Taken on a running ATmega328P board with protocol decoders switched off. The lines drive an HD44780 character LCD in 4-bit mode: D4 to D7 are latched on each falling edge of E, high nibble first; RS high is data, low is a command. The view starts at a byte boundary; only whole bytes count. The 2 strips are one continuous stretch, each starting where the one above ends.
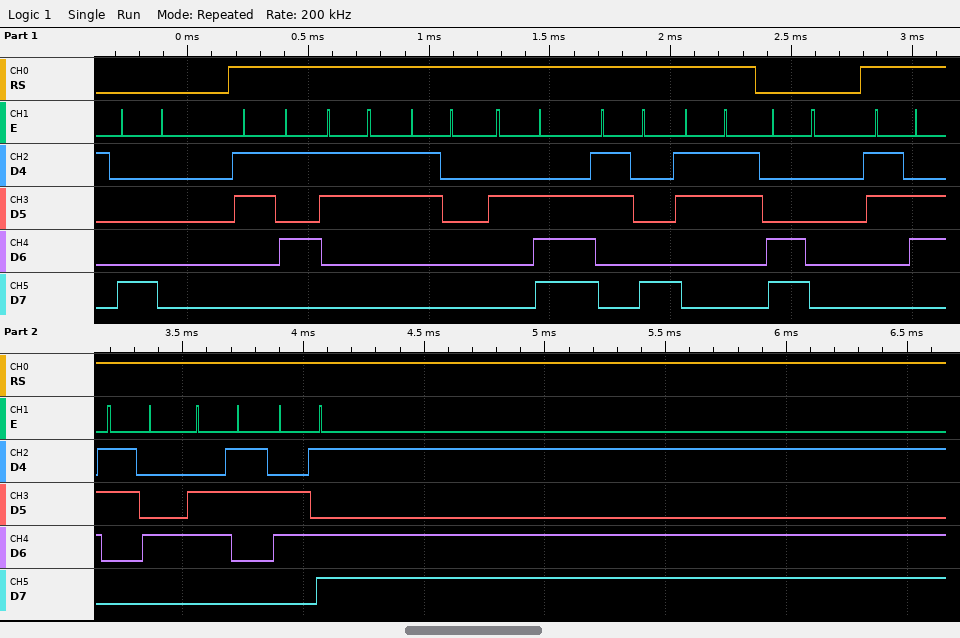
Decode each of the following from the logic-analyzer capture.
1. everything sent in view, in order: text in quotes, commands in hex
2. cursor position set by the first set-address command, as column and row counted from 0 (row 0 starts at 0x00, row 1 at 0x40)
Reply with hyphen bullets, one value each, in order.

- 0x80 "530.83" 0xC0 "64cm"
- column 0, row 0
